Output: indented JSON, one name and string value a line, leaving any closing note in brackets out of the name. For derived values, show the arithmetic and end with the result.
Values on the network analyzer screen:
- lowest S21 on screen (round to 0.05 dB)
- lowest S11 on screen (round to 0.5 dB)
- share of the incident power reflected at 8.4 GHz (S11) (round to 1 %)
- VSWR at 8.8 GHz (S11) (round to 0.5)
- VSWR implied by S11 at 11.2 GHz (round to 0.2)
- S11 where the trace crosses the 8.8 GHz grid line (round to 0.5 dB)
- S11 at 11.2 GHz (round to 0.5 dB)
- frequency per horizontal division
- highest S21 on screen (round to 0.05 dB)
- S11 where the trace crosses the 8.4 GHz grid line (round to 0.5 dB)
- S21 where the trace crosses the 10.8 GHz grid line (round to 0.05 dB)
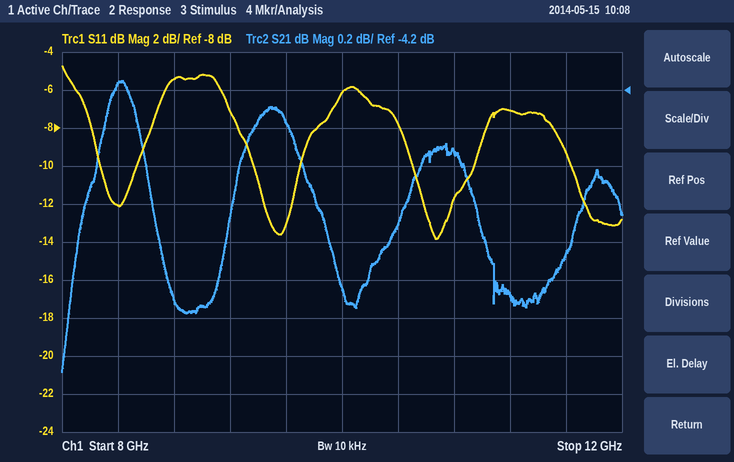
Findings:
{
  "lowest S21 on screen": "-5.70 dB",
  "lowest S11 on screen": "-14.0 dB",
  "share of the incident power reflected at 8.4 GHz (S11)": "10^(-12/10) ≈ 6 %",
  "VSWR at 8.8 GHz (S11)": "|Γ| = 10^(-5.5/20) = 0.5309; VSWR = (1 + 0.5309)/(1 − 0.5309) ≈ 3.26, so 3.5 to the nearest 0.5",
  "VSWR implied by S11 at 11.2 GHz": "|Γ| = 10^(-7/20) = 0.4467; VSWR = (1 + 0.4467)/(1 − 0.4467) ≈ 2.6",
  "S11 where the trace crosses the 8.8 GHz grid line": "-5.5 dB",
  "S11 at 11.2 GHz": "-7.0 dB",
  "frequency per horizontal division": "400 MHz",
  "highest S21 on screen": "-4.15 dB",
  "S11 where the trace crosses the 8.4 GHz grid line": "-12.0 dB",
  "S21 where the trace crosses the 10.8 GHz grid line": "-4.55 dB"
}
